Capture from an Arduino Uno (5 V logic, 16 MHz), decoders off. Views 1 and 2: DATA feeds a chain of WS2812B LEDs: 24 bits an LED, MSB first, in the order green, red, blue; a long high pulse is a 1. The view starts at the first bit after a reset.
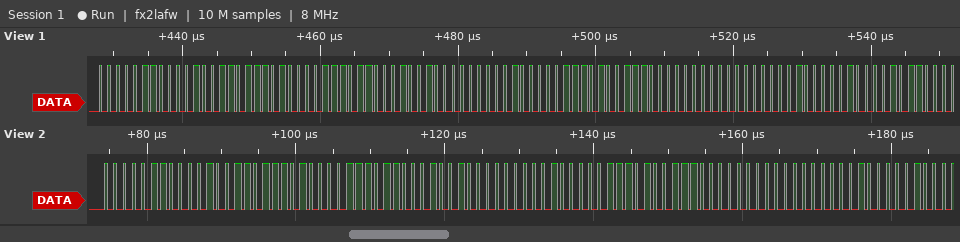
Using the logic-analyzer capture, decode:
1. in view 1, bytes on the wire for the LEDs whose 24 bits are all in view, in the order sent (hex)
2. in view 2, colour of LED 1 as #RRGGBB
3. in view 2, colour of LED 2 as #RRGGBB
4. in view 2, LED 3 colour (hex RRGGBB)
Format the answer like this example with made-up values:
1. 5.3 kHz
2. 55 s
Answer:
1. 06 13 74 3B 12 00 83 A7 00 00 41 0B
2. #130674
3. #123B00
4. #A78300
